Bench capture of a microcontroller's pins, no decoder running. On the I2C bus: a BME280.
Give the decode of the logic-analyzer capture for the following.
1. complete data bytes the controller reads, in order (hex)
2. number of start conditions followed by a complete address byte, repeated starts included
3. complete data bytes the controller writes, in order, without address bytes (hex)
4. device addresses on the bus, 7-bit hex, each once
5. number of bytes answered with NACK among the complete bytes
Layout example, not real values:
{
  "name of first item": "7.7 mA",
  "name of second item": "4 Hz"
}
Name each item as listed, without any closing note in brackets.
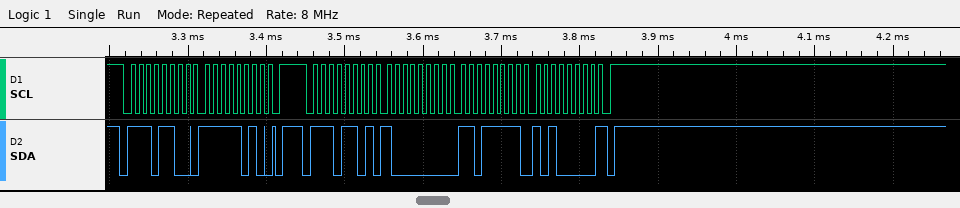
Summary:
{
  "complete data bytes the controller reads, in order": "80 DF A0",
  "number of start conditions followed by a complete address byte, repeated starts included": "2",
  "complete data bytes the controller writes, in order, without address bytes": "FA",
  "device addresses on the bus, 7-bit hex, each once": "0x76",
  "number of bytes answered with NACK among the complete bytes": "1"
}
